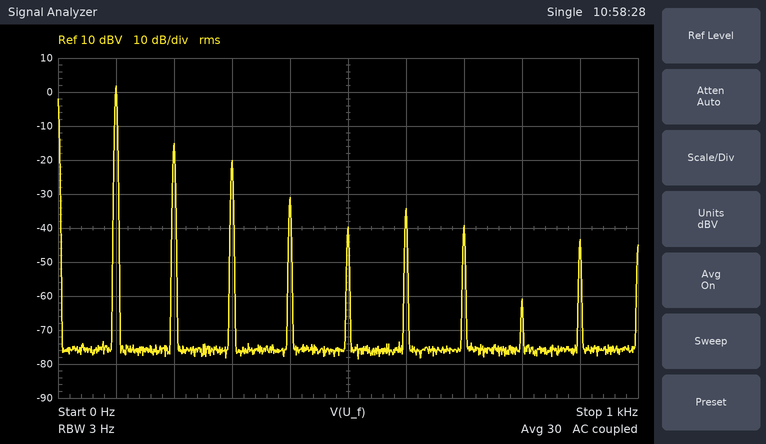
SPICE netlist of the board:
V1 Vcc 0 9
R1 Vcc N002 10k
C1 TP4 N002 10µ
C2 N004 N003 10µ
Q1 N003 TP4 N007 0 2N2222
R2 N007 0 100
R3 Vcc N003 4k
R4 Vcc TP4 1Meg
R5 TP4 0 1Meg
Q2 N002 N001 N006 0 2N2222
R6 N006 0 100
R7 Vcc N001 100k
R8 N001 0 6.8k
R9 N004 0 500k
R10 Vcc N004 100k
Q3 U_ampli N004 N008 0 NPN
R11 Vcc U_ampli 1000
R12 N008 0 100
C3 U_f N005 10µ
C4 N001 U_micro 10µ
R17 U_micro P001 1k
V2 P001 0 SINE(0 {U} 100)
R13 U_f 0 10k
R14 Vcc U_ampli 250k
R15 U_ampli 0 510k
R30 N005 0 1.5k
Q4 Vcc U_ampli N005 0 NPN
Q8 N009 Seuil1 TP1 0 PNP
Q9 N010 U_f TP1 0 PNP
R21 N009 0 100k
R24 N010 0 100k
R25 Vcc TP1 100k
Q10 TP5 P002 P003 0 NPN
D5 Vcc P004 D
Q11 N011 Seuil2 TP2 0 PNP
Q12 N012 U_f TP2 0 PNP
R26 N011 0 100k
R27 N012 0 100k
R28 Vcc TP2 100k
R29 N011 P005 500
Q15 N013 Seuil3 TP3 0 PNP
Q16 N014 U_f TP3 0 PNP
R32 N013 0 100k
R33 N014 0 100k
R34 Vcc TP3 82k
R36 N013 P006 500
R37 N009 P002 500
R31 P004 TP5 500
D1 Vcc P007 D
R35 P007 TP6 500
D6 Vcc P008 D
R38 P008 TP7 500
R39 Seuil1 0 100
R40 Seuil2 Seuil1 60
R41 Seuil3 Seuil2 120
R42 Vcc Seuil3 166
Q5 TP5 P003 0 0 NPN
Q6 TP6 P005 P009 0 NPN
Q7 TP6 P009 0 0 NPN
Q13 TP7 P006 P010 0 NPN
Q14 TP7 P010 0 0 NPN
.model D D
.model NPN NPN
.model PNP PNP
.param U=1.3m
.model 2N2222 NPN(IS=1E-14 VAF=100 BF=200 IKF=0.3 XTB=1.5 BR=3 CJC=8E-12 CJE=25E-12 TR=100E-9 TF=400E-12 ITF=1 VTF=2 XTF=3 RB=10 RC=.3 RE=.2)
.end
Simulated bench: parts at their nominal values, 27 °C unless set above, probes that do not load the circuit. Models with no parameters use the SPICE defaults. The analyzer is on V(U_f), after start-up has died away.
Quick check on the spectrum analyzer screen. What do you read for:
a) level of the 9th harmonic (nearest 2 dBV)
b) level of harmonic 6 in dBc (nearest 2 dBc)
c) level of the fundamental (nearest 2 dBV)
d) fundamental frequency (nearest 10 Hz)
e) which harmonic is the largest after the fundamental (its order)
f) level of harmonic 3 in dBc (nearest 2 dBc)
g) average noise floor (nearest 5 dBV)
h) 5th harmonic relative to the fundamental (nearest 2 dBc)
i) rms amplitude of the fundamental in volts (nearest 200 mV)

-44 dBV
-36 dBc
2 dBV
100 Hz
2
-22 dBc
-75 dBV
-42 dBc
1.2 V
